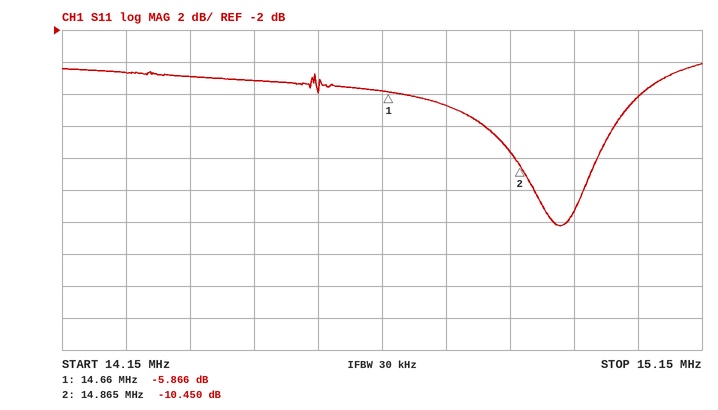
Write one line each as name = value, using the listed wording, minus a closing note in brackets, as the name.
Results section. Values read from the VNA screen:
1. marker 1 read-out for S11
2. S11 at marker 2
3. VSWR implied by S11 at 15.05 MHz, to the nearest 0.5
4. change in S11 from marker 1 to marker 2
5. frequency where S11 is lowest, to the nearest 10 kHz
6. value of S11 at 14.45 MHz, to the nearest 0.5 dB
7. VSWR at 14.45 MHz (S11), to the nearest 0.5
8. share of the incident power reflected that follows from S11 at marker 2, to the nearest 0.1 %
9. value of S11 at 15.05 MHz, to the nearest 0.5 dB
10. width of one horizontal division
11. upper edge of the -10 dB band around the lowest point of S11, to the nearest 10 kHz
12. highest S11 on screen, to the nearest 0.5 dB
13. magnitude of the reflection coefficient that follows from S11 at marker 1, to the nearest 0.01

marker 1 read-out for S11 = -5.866 dB
S11 at marker 2 = -10.450 dB
VSWR implied by S11 at 15.05 MHz, to the nearest 0.5 = 3.0
change in S11 from marker 1 to marker 2 = -4.584 dB
frequency where S11 is lowest, to the nearest 10 kHz = 14.93 MHz
value of S11 at 14.45 MHz, to the nearest 0.5 dB = -5.0 dB
VSWR at 14.45 MHz (S11), to the nearest 0.5 = 3.5
share of the incident power reflected that follows from S11 at marker 2, to the nearest 0.1 % = 9.0 %
value of S11 at 15.05 MHz, to the nearest 0.5 dB = -6.0 dB
width of one horizontal division = 100 kHz
upper edge of the -10 dB band around the lowest point of S11, to the nearest 10 kHz = 14.99 MHz
highest S11 on screen, to the nearest 0.5 dB = -4.0 dB
magnitude of the reflection coefficient that follows from S11 at marker 1, to the nearest 0.01 = 0.51
